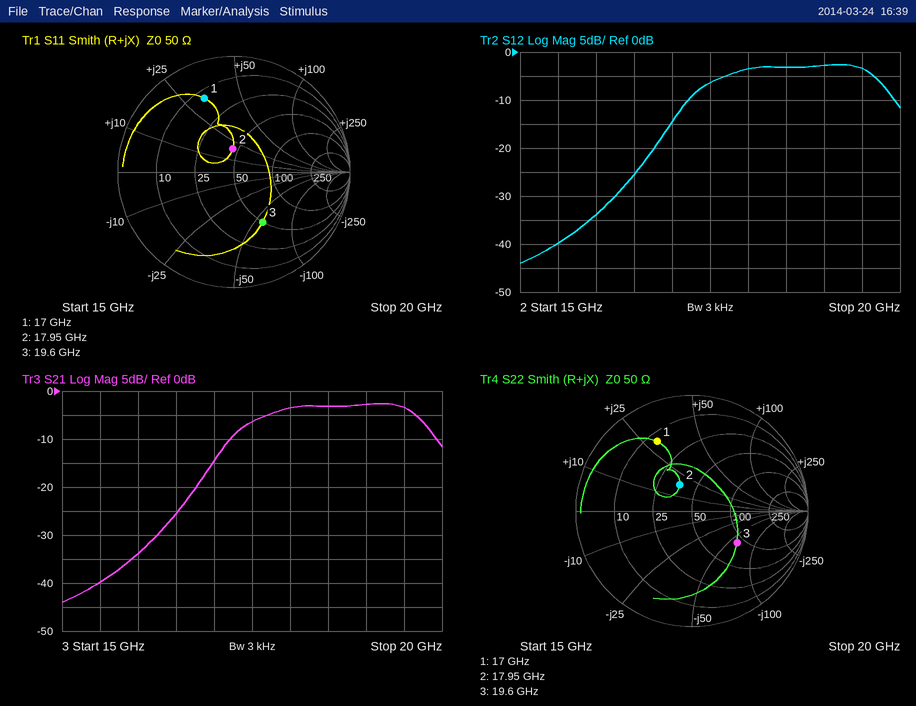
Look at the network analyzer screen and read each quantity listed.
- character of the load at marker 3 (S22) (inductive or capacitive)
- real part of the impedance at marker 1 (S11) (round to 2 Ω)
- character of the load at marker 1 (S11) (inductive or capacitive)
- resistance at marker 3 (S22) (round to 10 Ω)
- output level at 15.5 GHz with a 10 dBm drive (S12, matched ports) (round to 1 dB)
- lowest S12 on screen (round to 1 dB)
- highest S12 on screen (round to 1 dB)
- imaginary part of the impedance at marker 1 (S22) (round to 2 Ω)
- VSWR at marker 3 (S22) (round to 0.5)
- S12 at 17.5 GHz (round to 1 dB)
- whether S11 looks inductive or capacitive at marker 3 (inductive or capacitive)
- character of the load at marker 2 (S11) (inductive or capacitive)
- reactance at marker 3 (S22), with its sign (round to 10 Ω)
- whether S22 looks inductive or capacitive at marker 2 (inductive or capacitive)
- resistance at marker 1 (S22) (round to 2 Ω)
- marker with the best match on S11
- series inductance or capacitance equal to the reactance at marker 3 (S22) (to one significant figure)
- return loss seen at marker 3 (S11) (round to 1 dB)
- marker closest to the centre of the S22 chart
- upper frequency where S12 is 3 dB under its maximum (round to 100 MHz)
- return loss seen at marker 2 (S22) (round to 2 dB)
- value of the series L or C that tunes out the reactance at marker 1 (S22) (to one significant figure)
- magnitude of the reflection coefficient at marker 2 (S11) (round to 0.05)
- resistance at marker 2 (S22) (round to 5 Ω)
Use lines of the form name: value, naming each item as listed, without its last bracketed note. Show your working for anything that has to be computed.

character of the load at marker 3 (S22): capacitive
real part of the impedance at marker 1 (S11): 14 Ω
character of the load at marker 1 (S11): inductive
resistance at marker 3 (S22): 90 Ω
output level at 15.5 GHz with a 10 dBm drive (S12, matched ports): 10 dBm + (-40 dB) = -30 dBm
lowest S12 on screen: -44 dB
highest S12 on screen: -3 dB
imaginary part of the impedance at marker 1 (S22): +30 Ω
VSWR at marker 3 (S22): 3.0
S12 at 17.5 GHz: -6 dB
whether S11 looks inductive or capacitive at marker 3: capacitive
character of the load at marker 2 (S11): inductive
reactance at marker 3 (S22), with its sign: -60 Ω
whether S22 looks inductive or capacitive at marker 2: inductive
resistance at marker 1 (S22): 14 Ω
marker with the best match on S11: marker 2
series inductance or capacitance equal to the reactance at marker 3 (S22): C = 1/(2π × 19.6 GHz × 60 Ω) ≈ 135 fF, so 100 fF to one significant figure
return loss seen at marker 3 (S11): 6 dB
marker closest to the centre of the S22 chart: marker 2
upper frequency where S12 is 3 dB under its maximum: 19.7 GHz
return loss seen at marker 2 (S22): 12 dB
value of the series L or C that tunes out the reactance at marker 1 (S22): C = 1/(2π × 17 GHz × 30 Ω) ≈ 312 fF, so 300 fF to one significant figure
magnitude of the reflection coefficient at marker 2 (S11): 0.20
resistance at marker 2 (S22): 35 Ω
